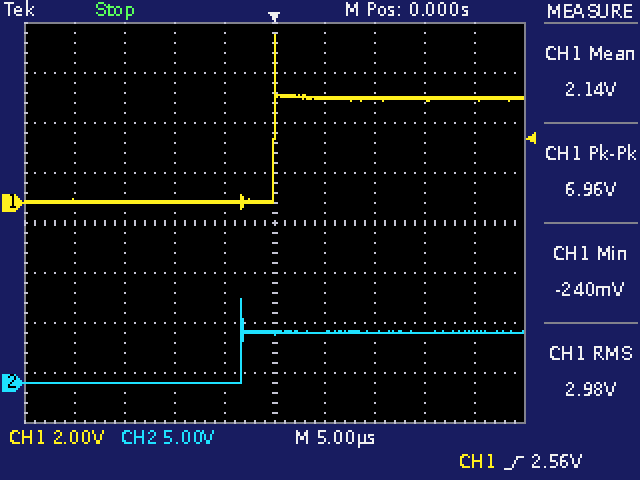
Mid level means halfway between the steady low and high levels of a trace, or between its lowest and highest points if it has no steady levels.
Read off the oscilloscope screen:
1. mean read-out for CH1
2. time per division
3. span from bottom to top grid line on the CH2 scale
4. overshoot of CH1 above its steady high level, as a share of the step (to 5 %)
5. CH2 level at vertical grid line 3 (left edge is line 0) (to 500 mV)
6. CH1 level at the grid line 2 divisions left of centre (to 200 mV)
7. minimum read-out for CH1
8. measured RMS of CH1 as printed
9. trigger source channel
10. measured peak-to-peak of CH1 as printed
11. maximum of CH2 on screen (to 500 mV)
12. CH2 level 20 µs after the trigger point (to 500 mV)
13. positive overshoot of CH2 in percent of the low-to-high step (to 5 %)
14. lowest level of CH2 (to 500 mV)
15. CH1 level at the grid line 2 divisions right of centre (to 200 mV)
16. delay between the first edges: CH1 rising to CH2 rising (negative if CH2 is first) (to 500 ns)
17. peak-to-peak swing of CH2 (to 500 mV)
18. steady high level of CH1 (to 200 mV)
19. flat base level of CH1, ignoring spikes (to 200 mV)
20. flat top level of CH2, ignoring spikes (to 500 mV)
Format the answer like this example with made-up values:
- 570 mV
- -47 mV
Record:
- 2.14 V
- 5 µs
- 40 V
- 60 %
- 0.0 V
- 0.0 V
- -240 mV
- 2.98 V
- CH1
- 6.96 V
- 8.5 V
- 5.0 V
- 70 %
- 0.0 V
- 4.2 V
- -3.5 µs
- 8.5 V
- 4.2 V
- 0.0 V
- 5.0 V
